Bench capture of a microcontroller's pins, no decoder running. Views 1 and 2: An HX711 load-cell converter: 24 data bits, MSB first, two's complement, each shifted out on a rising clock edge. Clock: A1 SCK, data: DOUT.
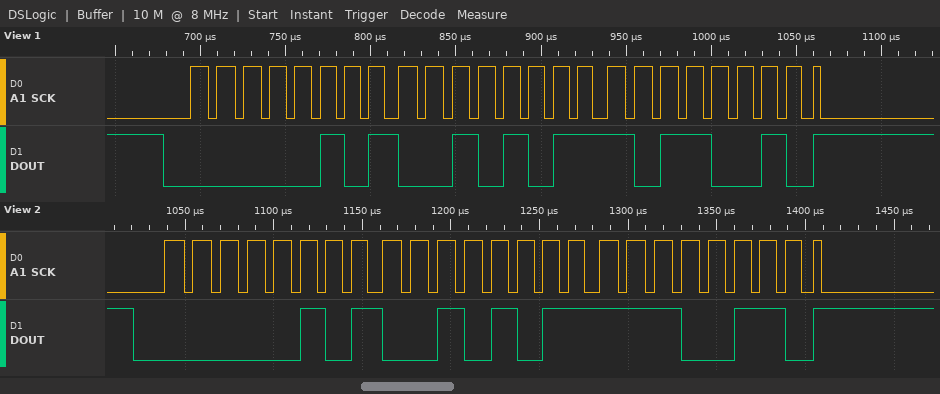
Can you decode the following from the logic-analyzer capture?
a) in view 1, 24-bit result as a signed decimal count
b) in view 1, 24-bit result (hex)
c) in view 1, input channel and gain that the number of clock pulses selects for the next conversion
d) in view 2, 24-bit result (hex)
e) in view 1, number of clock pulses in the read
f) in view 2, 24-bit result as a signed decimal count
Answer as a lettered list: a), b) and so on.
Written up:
a) 338866
b) 0x052BB2
c) channel A, gain 128
d) 0x052BE6
e) 25
f) 338918
